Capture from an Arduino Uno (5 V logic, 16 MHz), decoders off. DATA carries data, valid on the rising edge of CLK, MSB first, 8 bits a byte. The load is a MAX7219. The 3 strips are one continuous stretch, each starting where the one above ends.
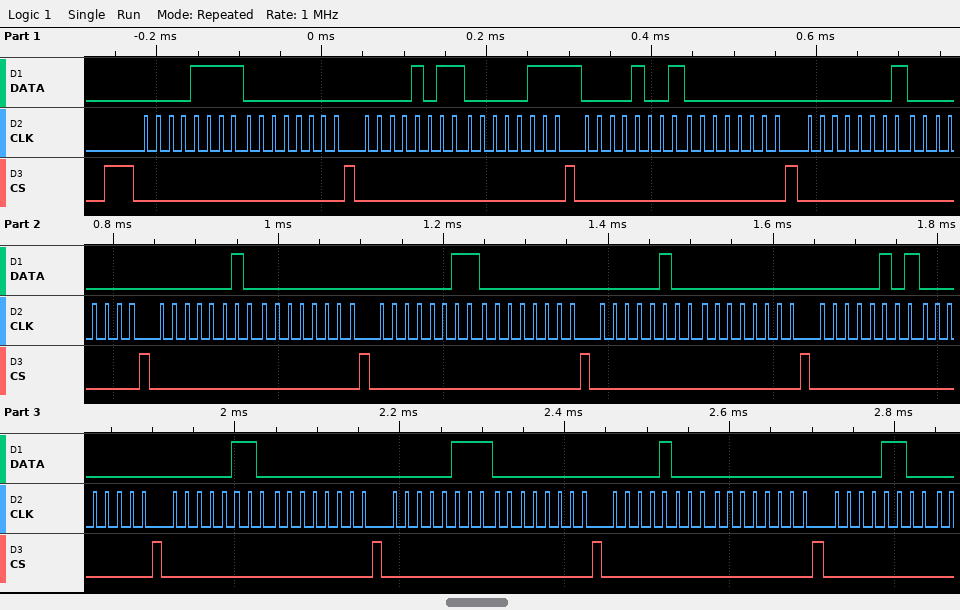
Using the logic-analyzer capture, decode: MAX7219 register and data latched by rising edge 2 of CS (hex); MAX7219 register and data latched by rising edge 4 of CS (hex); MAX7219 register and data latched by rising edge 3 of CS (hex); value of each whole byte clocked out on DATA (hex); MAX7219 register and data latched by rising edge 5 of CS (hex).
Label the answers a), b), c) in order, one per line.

a) register 0xF, data 0x00
b) register 0x9, data 0x00
c) register 0xB, data 0x07
d) 0x0F 0x00 0x0B 0x07 0x09 0x00 0x01 0x00 0x02 0x00 0x03 0x00 0x04 0x00 0x05 0x00 0x06 0x00 0x07 0x00 0x08 0x00 0x0C
e) register 0x1, data 0x00
